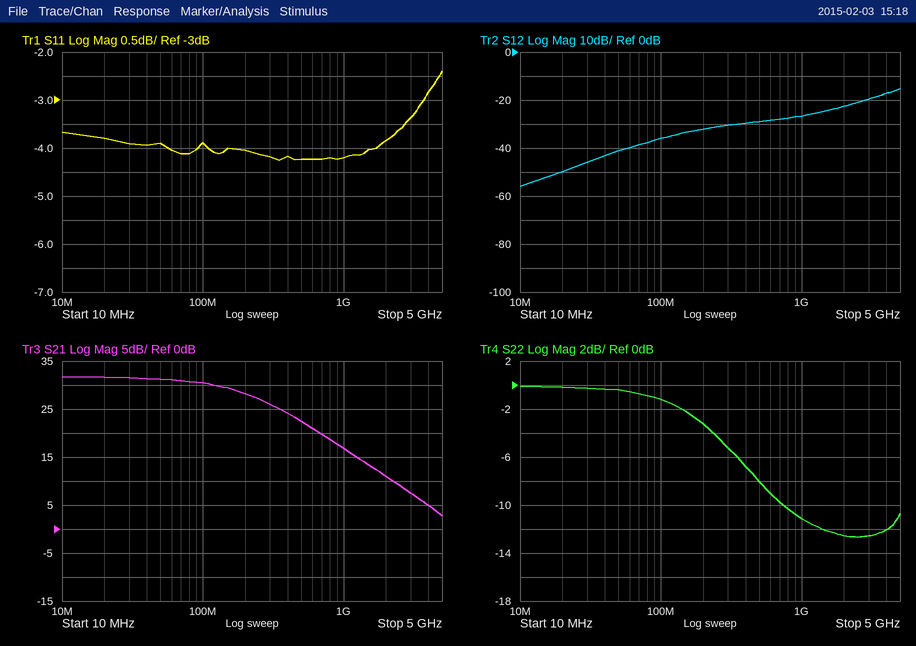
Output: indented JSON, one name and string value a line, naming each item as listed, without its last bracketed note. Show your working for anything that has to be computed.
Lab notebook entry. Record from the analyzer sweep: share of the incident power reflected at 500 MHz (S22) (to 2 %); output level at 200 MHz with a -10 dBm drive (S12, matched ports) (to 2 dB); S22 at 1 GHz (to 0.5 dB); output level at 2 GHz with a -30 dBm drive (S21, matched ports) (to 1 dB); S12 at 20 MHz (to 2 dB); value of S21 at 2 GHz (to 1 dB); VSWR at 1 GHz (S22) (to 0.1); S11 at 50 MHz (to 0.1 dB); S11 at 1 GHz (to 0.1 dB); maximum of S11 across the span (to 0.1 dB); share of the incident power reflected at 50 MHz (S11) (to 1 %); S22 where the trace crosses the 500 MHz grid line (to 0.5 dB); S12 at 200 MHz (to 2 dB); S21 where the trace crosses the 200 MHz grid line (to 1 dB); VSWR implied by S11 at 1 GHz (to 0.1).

{
  "share of the incident power reflected at 500 MHz (S22)": "10^(-8/10) ≈ 16 %",
  "output level at 200 MHz with a -10 dBm drive (S12, matched ports)": "-10 dBm + (-32 dB) = -42 dBm",
  "S22 at 1 GHz": "-11.0 dB",
  "output level at 2 GHz with a -30 dBm drive (S21, matched ports)": "-30 dBm + (11 dB) = -19 dBm",
  "S12 at 20 MHz": "-50 dB",
  "value of S21 at 2 GHz": "11 dB",
  "VSWR at 1 GHz (S22)": "|Γ| = 10^(-11/20) = 0.2818; VSWR = (1 + 0.2818)/(1 − 0.2818) ≈ 1.8",
  "S11 at 50 MHz": "-3.9 dB",
  "S11 at 1 GHz": "-4.2 dB",
  "maximum of S11 across the span": "-2.4 dB",
  "share of the incident power reflected at 50 MHz (S11)": "10^(-3.9/10) ≈ 41 %",
  "S22 where the trace crosses the 500 MHz grid line": "-8.0 dB",
  "S12 at 200 MHz": "-32 dB",
  "S21 where the trace crosses the 200 MHz grid line": "28 dB",
  "VSWR implied by S11 at 1 GHz": "|Γ| = 10^(-4.2/20) = 0.6166; VSWR = (1 + 0.6166)/(1 − 0.6166) ≈ 4.2"
}
